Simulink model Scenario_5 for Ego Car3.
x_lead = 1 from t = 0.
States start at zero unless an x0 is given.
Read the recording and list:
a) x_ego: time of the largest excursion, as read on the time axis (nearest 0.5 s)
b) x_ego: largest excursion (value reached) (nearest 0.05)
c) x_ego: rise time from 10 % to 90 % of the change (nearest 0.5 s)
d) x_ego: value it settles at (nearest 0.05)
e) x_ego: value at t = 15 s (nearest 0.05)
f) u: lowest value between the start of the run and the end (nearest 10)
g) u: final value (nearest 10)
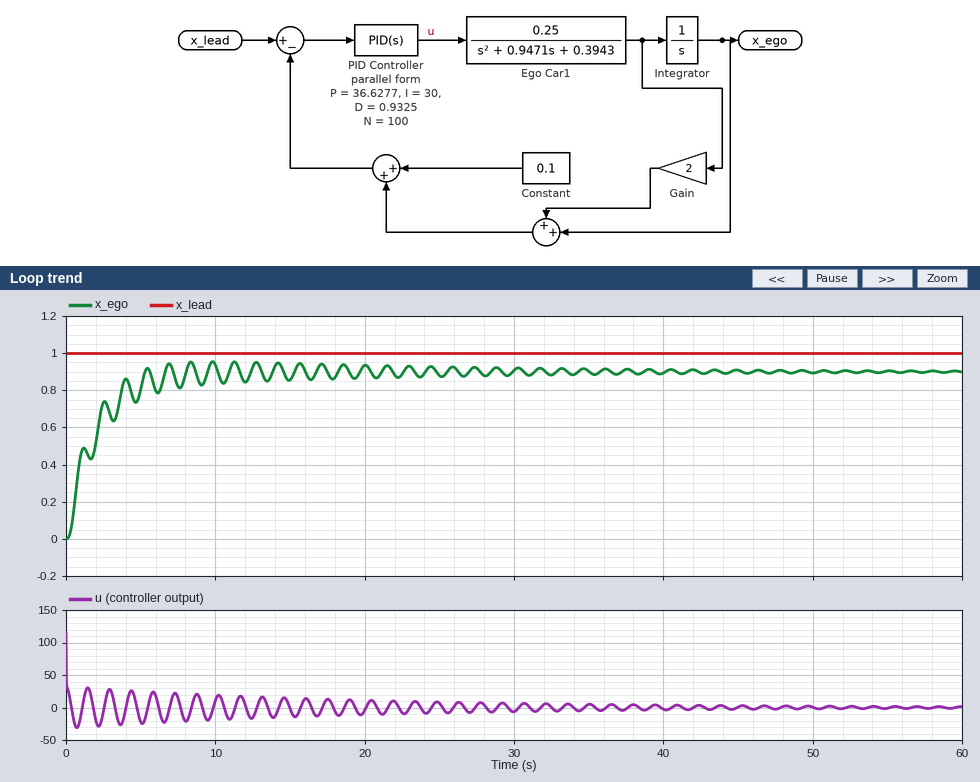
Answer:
10.0 s
0.95
3.5 s
0.90
0.85
-30
0
